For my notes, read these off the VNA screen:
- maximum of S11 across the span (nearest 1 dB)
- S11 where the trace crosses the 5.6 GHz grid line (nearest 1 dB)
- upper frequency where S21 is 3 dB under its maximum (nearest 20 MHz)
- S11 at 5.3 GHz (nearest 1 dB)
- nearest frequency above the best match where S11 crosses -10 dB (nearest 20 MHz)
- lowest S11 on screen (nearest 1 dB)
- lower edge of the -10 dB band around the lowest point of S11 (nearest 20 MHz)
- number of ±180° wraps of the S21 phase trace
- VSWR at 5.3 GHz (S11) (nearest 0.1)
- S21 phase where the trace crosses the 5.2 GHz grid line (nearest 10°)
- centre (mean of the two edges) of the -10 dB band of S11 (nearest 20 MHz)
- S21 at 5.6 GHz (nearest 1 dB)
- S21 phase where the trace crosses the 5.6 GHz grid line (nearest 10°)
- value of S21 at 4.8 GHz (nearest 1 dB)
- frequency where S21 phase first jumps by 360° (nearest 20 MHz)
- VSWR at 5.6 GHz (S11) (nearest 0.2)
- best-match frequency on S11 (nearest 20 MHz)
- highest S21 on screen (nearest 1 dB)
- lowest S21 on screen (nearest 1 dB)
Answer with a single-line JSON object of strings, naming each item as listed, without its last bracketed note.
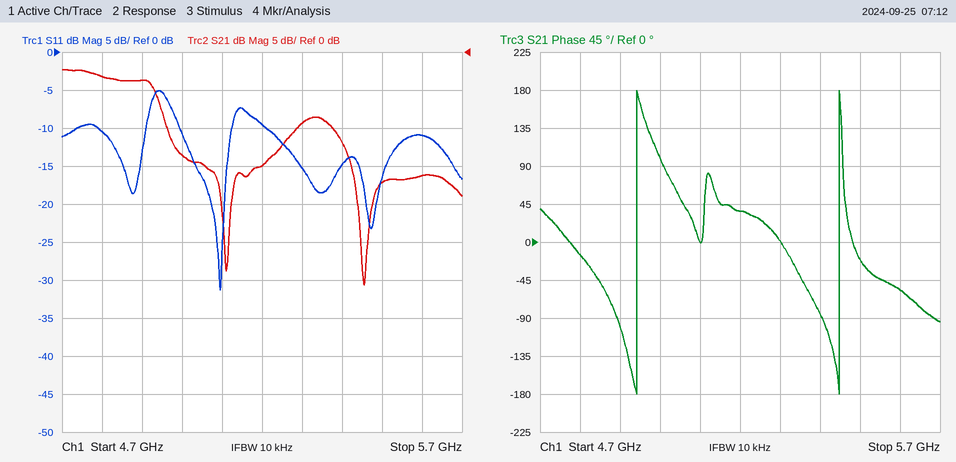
{"maximum of S11 across the span": "-5 dB", "S11 where the trace crosses the 5.6 GHz grid line": "-11 dB", "upper frequency where S21 is 3 dB under its maximum": "4.94 GHz", "S11 at 5.3 GHz": "-15 dB", "nearest frequency above the best match where S11 crosses -10 dB": "5.12 GHz", "lowest S11 on screen": "-31 dB", "lower edge of the -10 dB band around the lowest point of S11": "5.00 GHz", "number of ±180° wraps of the S21 phase trace": "2", "VSWR at 5.3 GHz (S11)": "1.4", "S21 phase where the trace crosses the 5.2 GHz grid line": "40°", "centre (mean of the two edges) of the -10 dB band of S11": "5.06 GHz", "S21 at 5.6 GHz": "-16 dB", "S21 phase where the trace crosses the 5.6 GHz grid line": "-60°", "value of S21 at 4.8 GHz": "-3 dB", "frequency where S21 phase first jumps by 360°": "4.94 GHz", "VSWR at 5.6 GHz (S11)": "1.8", "best-match frequency on S11": "5.10 GHz", "highest S21 on screen": "-2 dB", "lowest S21 on screen": "-31 dB"}
